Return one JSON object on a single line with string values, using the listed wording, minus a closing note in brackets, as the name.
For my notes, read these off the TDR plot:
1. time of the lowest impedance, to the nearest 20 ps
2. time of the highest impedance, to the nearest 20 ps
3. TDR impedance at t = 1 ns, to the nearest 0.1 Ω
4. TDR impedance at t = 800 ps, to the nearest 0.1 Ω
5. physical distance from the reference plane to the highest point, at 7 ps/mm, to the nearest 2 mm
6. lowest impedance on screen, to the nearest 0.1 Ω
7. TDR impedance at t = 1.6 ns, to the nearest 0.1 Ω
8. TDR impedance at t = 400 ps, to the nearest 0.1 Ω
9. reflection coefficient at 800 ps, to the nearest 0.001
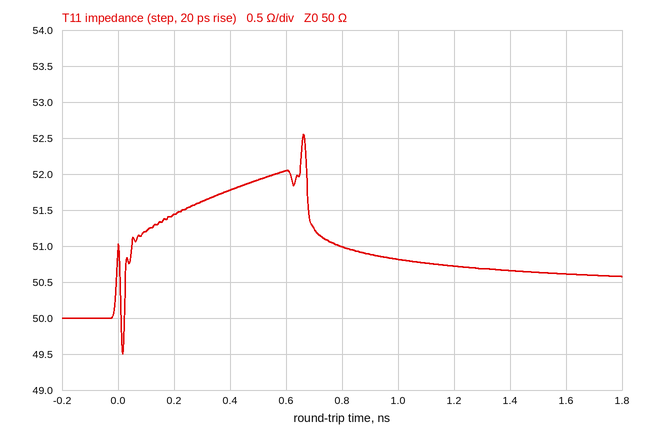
{"time of the lowest impedance, to the nearest 20 ps": "20 ps", "time of the highest impedance, to the nearest 20 ps": "660 ps", "TDR impedance at t = 1 ns, to the nearest 0.1 Ω": "50.8 Ω", "TDR impedance at t = 800 ps, to the nearest 0.1 Ω": "51.0 Ω", "physical distance from the reference plane to the highest point, at 7 ps/mm, to the nearest 2 mm": "48 mm", "lowest impedance on screen, to the nearest 0.1 Ω": "49.5 Ω", "TDR impedance at t = 1.6 ns, to the nearest 0.1 Ω": "50.6 Ω", "TDR impedance at t = 400 ps, to the nearest 0.1 Ω": "51.8 Ω", "reflection coefficient at 800 ps, to the nearest 0.001": "+0.010"}
